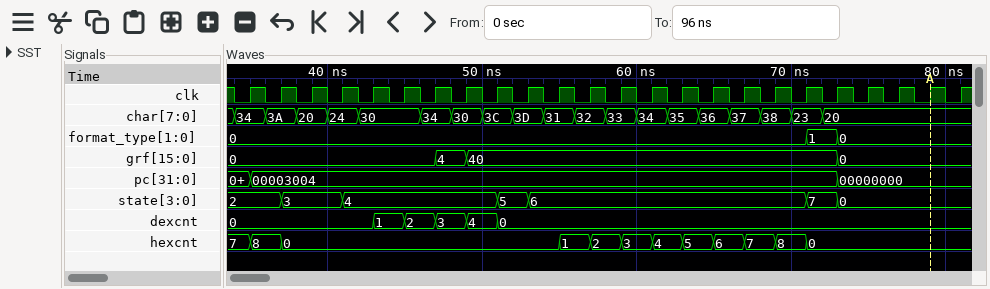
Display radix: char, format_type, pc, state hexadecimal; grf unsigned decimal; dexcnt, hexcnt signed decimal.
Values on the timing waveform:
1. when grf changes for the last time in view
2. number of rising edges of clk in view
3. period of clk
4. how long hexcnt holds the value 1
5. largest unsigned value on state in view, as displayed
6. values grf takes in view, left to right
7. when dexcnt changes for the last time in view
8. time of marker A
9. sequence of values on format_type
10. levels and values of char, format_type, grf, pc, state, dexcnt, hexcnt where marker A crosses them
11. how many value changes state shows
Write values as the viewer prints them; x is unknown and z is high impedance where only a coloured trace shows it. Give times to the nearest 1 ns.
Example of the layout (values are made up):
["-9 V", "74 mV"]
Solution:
["73 ns", "24", "2 ns", "2 ns", "7", "0, 4, 40, 0", "51 ns", "79 ns", "0, 1, 0", "char=20, format_type=0, grf=0, pc=00000000, state=0, dexcnt=0, hexcnt=0", "6"]
